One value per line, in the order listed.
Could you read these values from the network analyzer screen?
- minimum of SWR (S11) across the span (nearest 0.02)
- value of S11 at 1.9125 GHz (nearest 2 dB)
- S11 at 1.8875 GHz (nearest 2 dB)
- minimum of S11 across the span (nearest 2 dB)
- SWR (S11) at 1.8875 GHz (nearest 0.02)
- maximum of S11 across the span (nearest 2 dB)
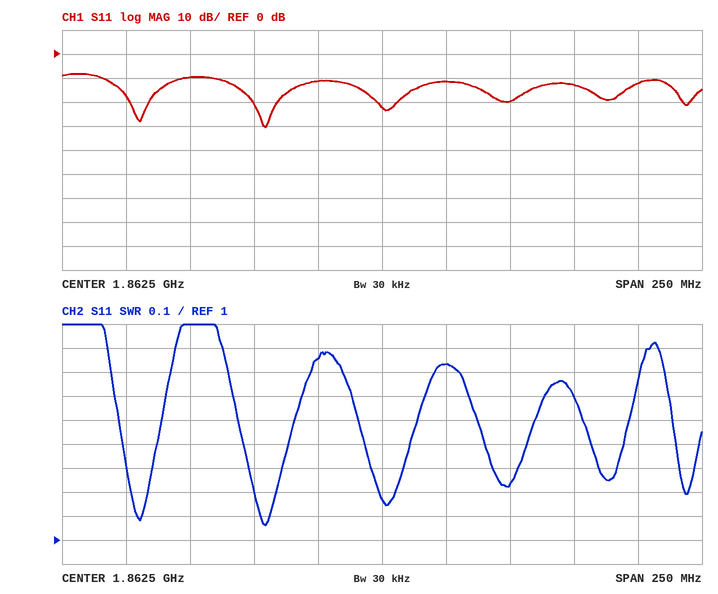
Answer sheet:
1.06
-20 dB
-12 dB
-30 dB
1.74
-8 dB
